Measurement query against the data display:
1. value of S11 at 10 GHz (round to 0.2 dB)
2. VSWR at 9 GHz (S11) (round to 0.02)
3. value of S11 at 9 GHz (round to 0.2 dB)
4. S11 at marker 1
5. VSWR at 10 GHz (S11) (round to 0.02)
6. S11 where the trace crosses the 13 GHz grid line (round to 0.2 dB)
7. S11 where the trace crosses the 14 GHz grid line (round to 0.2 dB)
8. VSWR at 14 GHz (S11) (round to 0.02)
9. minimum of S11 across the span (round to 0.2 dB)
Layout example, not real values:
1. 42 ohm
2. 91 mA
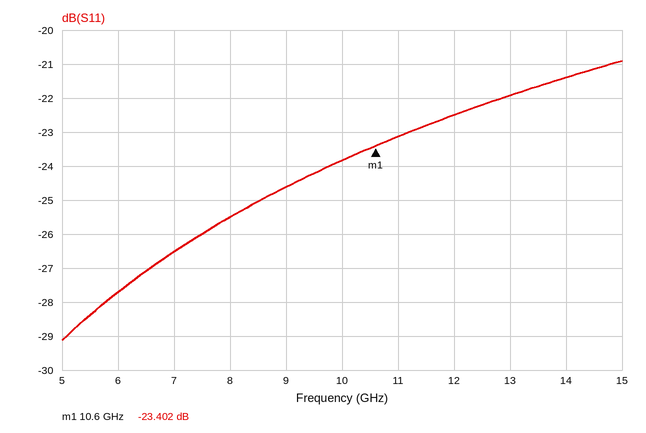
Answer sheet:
1. -23.8 dB
2. 1.12
3. -24.6 dB
4. -23.402 dB
5. 1.14
6. -22.0 dB
7. -21.4 dB
8. 1.18
9. -29.2 dB
